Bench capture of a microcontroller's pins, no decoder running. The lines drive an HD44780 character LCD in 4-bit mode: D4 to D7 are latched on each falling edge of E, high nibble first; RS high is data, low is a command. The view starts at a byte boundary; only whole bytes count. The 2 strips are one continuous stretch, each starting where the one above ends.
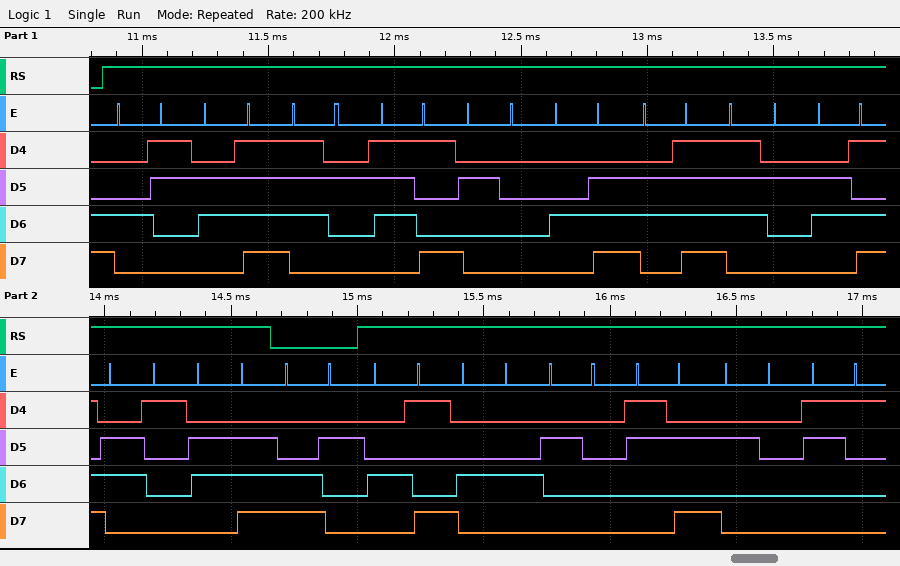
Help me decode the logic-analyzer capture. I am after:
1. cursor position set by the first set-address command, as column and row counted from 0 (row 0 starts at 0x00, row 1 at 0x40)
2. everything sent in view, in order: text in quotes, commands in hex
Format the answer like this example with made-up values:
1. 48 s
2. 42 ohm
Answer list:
1. column 2, row 1
2. "Cory Norman" 0xC2 "ID : 1"
